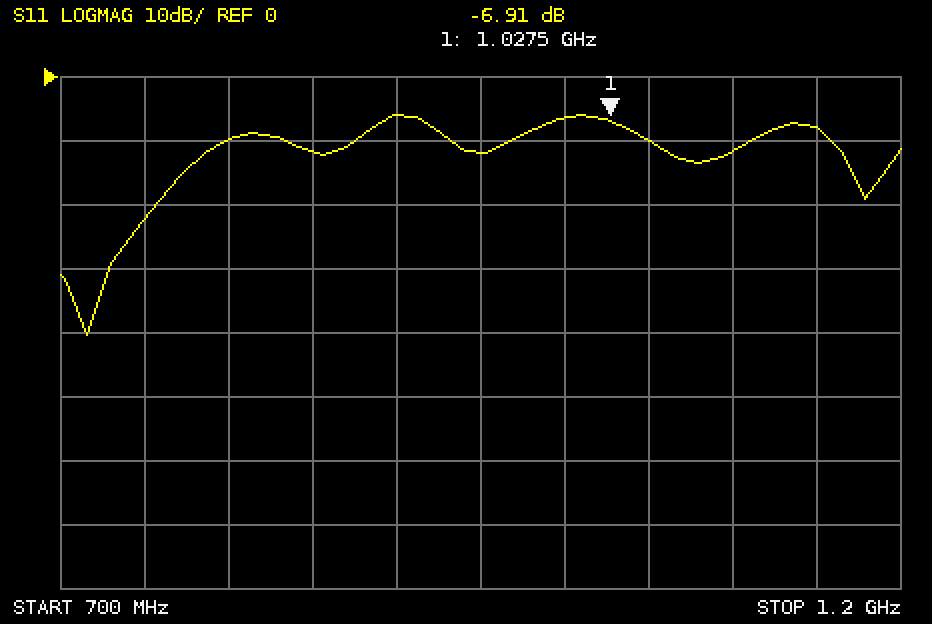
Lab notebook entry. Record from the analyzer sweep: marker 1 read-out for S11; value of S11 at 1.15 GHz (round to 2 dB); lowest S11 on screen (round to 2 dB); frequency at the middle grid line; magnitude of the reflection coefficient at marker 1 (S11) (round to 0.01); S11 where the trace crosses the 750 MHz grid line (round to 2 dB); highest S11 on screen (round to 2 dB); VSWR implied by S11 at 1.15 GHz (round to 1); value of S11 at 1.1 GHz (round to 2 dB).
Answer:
-6.91 dB
-8 dB
-40 dB
950 MHz
0.45
-22 dB
-6 dB
2
-12 dB
